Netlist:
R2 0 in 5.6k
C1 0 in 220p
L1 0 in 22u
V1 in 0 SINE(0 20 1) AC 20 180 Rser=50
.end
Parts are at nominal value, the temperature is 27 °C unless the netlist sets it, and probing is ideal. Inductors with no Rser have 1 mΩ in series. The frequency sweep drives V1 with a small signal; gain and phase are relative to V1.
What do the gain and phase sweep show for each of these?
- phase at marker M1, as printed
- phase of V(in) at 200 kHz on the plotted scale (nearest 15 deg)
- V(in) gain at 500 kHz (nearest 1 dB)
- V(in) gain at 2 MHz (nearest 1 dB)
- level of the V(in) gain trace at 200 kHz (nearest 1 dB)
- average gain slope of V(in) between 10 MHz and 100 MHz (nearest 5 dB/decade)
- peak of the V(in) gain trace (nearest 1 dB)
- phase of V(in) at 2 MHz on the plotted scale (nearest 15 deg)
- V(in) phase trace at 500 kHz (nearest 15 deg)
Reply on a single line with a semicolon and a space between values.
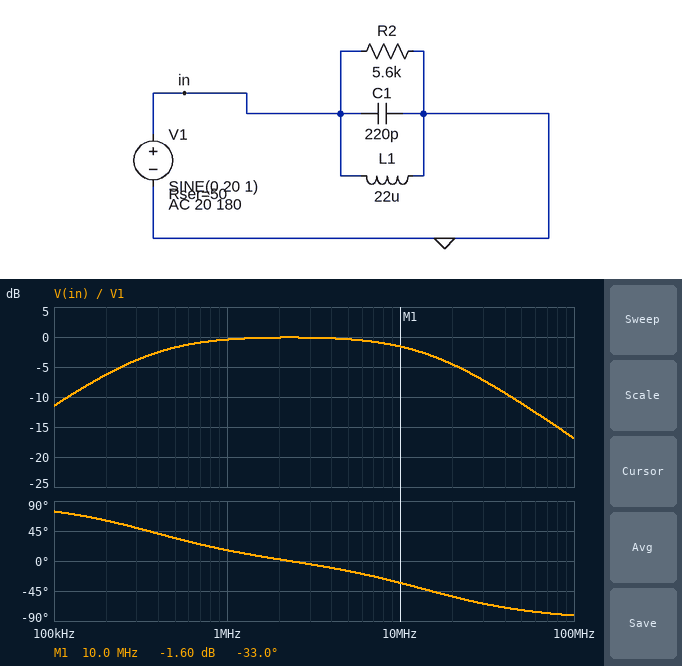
-33.0 deg; 60 deg; -2 dB; 0 dB; -6 dB; -15 dB/decade; 0 dB; 0 deg; 30 deg
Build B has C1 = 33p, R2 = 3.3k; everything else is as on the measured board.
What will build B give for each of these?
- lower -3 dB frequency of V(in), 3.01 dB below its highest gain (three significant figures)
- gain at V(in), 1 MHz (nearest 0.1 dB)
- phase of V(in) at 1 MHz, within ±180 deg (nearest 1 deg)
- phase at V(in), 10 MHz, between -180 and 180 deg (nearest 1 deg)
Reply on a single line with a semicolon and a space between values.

355 kHz; -0.6 dB; 19 deg; -4 deg
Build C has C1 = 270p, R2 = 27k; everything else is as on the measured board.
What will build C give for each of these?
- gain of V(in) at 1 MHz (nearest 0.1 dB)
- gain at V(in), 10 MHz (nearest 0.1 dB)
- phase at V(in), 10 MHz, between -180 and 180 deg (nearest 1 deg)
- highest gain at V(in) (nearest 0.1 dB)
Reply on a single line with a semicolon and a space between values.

-0.3 dB; -2.2 dB; -39 deg; 0 dB
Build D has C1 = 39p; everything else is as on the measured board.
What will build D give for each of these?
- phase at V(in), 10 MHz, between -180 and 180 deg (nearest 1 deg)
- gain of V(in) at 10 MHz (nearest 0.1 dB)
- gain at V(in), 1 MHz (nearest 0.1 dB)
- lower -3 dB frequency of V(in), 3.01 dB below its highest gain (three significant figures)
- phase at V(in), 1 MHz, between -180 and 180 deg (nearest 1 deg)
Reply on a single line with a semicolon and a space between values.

-5 deg; -0.1 dB; -0.6 dB; 357 kHz; 19 deg
